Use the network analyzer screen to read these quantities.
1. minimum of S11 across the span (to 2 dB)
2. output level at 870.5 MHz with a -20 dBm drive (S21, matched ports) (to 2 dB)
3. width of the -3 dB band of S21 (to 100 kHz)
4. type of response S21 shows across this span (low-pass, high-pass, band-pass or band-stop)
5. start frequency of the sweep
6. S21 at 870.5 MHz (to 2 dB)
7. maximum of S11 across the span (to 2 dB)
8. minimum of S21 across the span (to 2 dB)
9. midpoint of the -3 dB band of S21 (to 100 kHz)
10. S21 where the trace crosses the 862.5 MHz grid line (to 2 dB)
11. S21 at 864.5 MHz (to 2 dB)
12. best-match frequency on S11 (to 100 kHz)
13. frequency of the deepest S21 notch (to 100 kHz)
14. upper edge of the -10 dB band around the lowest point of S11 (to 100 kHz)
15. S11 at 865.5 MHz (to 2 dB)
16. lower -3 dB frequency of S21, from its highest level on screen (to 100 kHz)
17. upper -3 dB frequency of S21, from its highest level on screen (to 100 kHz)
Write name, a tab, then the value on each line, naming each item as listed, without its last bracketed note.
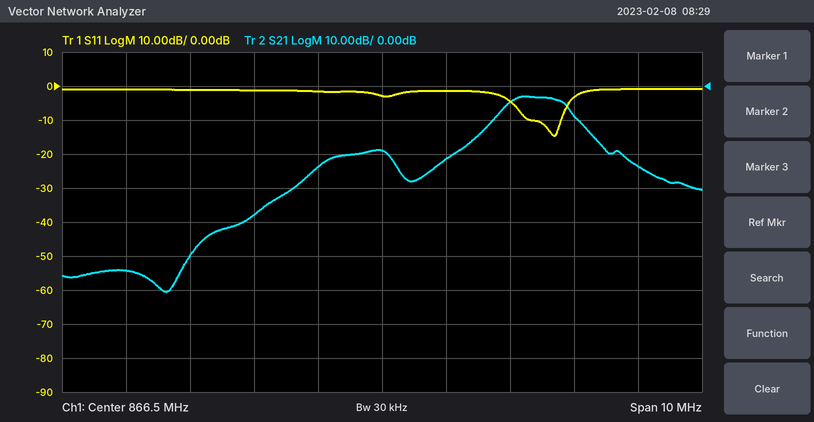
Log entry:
minimum of S11 across the span	-14 dB
output level at 870.5 MHz with a -20 dBm drive (S21, matched ports)	-44 dBm
width of the -3 dB band of S21	1.0 MHz
type of response S21 shows across this span	band-pass
start frequency of the sweep	861.5 MHz
S21 at 870.5 MHz	-24 dB
maximum of S11 across the span	0 dB
minimum of S21 across the span	-60 dB
midpoint of the -3 dB band of S21	868.9 MHz
S21 where the trace crosses the 862.5 MHz grid line	-54 dB
S21 at 864.5 MHz	-38 dB
best-match frequency on S11	869.2 MHz
frequency of the deepest S21 notch	863.1 MHz
upper edge of the -10 dB band around the lowest point of S11	869.3 MHz
S11 at 865.5 MHz	-2 dB
lower -3 dB frequency of S21, from its highest level on screen	868.4 MHz
upper -3 dB frequency of S21, from its highest level on screen	869.4 MHz
